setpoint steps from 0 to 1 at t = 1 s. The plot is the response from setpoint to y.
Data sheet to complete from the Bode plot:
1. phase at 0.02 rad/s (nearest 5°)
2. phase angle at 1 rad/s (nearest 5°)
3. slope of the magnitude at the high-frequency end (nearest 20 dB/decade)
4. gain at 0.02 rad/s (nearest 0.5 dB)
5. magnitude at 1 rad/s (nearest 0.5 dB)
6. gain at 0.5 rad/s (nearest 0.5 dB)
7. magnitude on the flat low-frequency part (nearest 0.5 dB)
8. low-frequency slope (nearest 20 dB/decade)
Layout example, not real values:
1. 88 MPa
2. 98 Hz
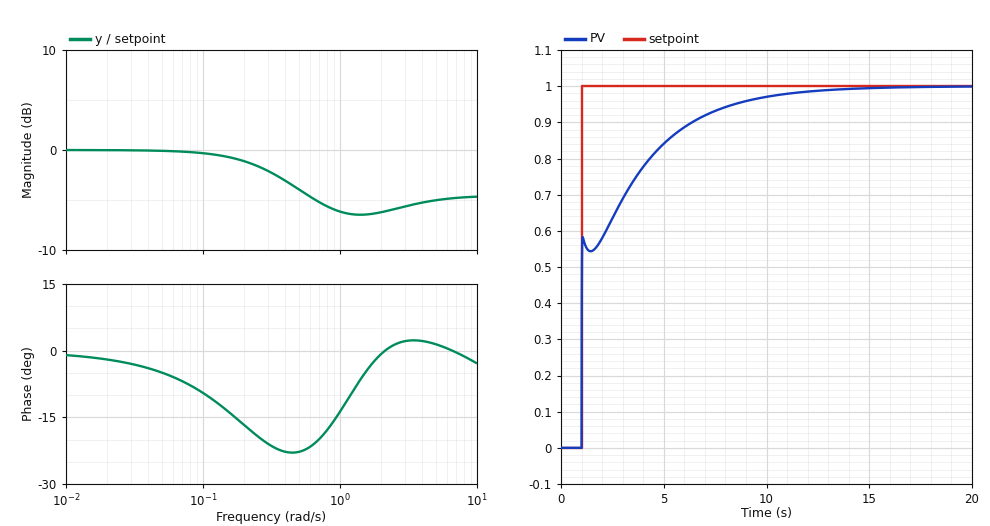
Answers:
1. 0°
2. -15°
3. 0 dB/decade
4. 0.0 dB
5. -6.0 dB
6. -4.0 dB
7. 0.0 dB
8. 0 dB/decade
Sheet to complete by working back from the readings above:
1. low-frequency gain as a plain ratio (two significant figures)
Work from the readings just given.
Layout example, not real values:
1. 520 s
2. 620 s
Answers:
1. 1.0
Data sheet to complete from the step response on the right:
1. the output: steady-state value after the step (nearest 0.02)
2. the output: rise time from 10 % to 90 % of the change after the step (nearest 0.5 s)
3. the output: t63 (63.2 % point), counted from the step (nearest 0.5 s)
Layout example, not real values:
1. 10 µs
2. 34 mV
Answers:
1. 1.00
2. 5.5 s
3. 1.5 s
